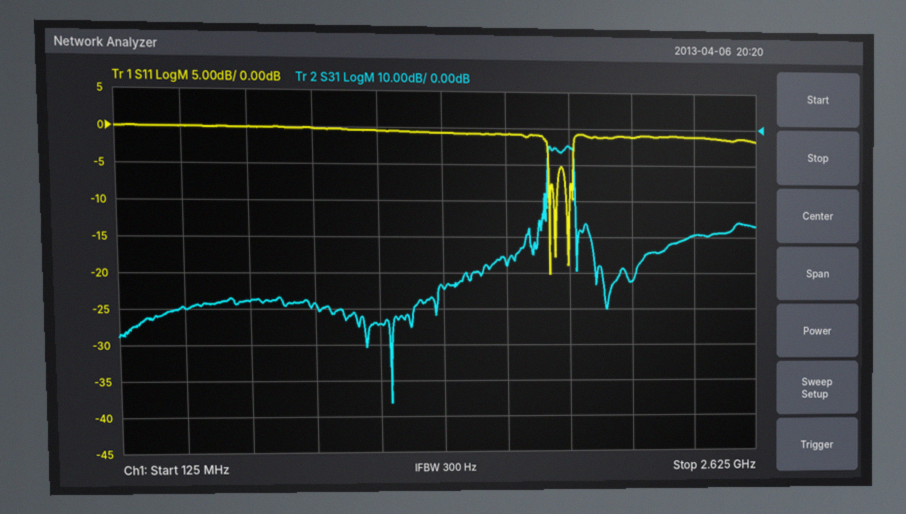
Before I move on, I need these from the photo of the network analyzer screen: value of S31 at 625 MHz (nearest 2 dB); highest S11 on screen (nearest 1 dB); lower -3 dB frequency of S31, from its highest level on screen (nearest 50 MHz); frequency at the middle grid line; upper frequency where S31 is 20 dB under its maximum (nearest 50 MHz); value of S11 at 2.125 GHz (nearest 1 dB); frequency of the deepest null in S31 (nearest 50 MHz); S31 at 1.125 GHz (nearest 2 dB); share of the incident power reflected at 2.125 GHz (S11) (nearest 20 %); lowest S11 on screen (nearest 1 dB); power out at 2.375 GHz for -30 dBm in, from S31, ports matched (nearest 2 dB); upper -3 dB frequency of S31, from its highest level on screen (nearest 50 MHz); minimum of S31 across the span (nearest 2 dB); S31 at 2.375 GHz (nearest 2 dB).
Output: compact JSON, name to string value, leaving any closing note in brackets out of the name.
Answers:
{"value of S31 at 625 MHz": "-48 dB", "highest S11 on screen": "0 dB", "lower -3 dB frequency of S31, from its highest level on screen": "1.80 GHz", "frequency at the middle grid line": "1.375 GHz", "upper frequency where S31 is 20 dB under its maximum": "1.90 GHz", "value of S11 at 2.125 GHz": "-1 dB", "frequency of the deepest null in S31": "1.15 GHz", "S31 at 1.125 GHz": "-54 dB", "share of the incident power reflected at 2.125 GHz (S11)": "80 %", "lowest S11 on screen": "-20 dB", "power out at 2.375 GHz for -30 dBm in, from S31, ports matched": "-60 dBm", "upper -3 dB frequency of S31, from its highest level on screen": "1.90 GHz", "minimum of S31 across the span": "-76 dB", "S31 at 2.375 GHz": "-30 dB"}
